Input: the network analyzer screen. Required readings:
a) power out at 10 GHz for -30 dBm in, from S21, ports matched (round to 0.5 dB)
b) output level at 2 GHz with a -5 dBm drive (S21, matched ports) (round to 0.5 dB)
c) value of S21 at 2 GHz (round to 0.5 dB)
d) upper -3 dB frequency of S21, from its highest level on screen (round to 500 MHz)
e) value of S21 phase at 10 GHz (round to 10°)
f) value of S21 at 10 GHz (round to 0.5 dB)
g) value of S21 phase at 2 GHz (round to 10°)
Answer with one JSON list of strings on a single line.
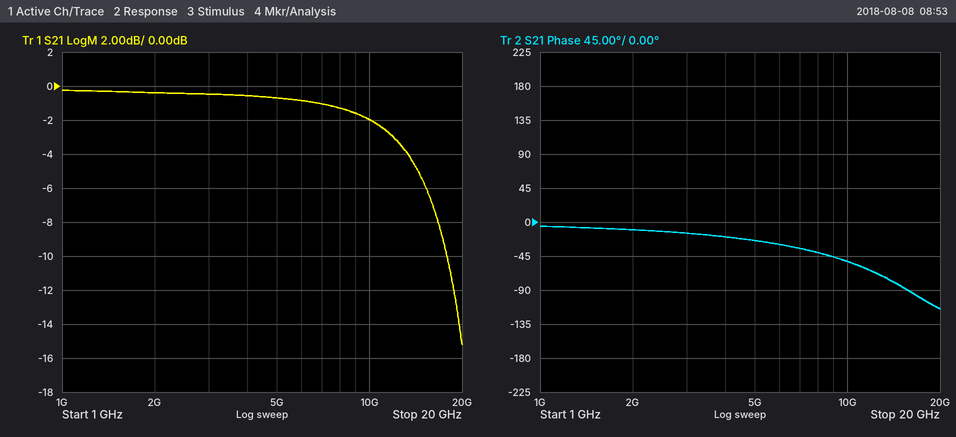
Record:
["-32.0 dBm", "-5.5 dBm", "-0.5 dB", "12.5 GHz", "-50°", "-2.0 dB", "-10°"]
